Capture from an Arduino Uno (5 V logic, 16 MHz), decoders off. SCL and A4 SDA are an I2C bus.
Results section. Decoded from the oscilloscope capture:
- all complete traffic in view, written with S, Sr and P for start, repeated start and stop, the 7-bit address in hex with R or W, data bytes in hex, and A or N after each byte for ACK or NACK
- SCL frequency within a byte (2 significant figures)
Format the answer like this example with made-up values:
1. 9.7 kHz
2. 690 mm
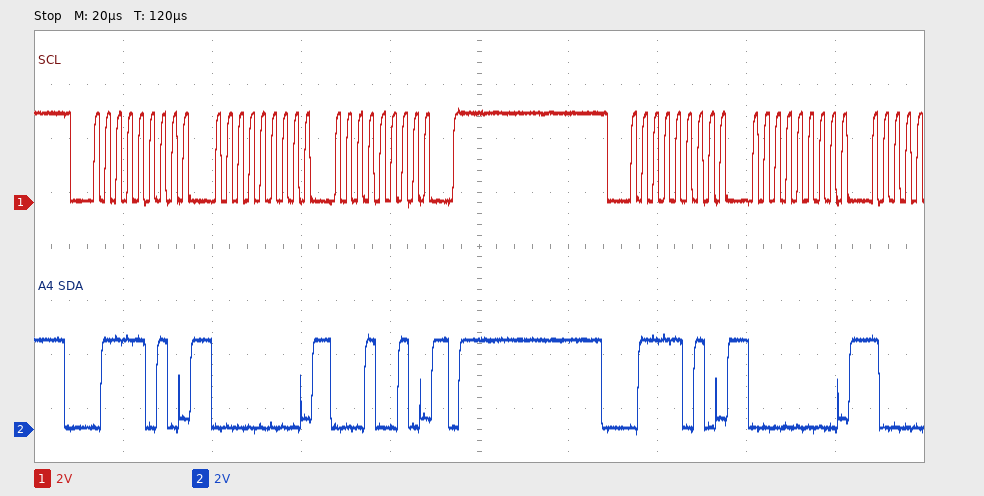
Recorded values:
1. S 3DW A 00 A 12 A P S 3DW A 00 A
2. 400 kHz
